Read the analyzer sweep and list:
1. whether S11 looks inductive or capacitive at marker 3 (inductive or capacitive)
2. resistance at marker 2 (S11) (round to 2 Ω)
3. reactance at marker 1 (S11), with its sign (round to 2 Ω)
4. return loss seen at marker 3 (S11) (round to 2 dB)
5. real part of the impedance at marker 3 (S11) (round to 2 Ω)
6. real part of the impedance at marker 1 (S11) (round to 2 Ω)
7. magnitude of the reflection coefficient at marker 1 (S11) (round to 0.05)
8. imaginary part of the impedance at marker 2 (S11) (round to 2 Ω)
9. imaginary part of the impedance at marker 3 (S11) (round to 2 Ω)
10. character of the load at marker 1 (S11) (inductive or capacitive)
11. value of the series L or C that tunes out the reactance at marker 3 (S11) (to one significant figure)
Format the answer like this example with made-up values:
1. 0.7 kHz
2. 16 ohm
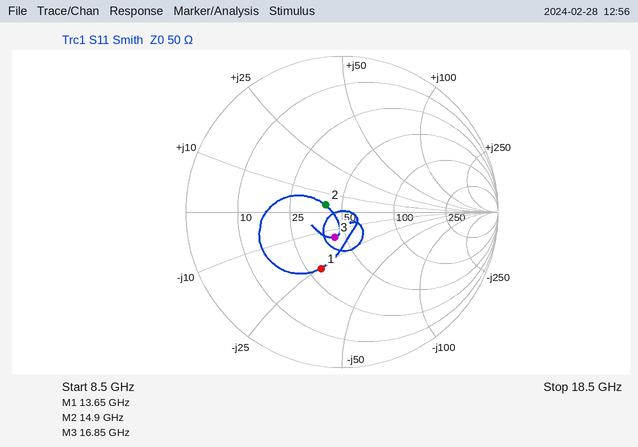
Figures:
1. capacitive
2. 40 Ω
3. -26 Ω
4. 16 dB
5. 44 Ω
6. 30 Ω
7. 0.40
8. +4 Ω
9. -14 Ω
10. capacitive
11. 100 pH
